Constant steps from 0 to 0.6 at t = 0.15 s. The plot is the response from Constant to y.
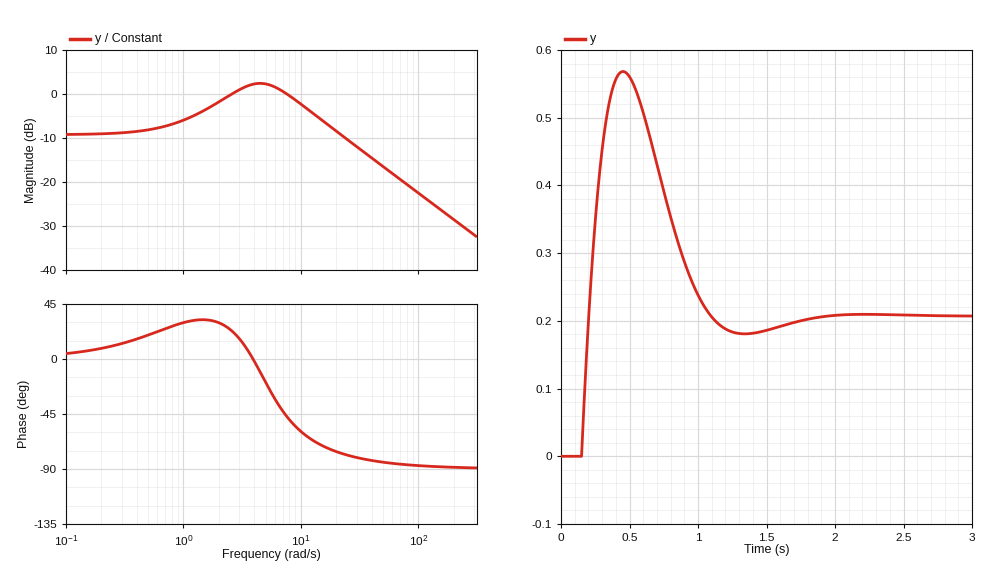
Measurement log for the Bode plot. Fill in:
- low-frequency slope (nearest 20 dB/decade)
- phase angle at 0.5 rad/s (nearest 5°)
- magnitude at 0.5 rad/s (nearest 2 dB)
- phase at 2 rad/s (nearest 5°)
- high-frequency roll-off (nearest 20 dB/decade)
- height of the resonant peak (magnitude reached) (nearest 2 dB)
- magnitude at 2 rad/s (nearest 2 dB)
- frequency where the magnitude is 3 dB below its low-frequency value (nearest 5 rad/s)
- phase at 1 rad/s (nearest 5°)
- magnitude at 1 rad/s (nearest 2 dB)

0 dB/decade
20°
-8 dB
30°
-20 dB/decade
2 dB
-2 dB
30 rad/s
30°
-6 dB
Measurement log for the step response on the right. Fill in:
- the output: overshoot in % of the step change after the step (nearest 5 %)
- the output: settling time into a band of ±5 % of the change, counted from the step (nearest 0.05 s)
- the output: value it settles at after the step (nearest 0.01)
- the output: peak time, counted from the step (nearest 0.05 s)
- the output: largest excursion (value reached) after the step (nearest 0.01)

175 %
1.55 s
0.21
0.30 s
0.57
